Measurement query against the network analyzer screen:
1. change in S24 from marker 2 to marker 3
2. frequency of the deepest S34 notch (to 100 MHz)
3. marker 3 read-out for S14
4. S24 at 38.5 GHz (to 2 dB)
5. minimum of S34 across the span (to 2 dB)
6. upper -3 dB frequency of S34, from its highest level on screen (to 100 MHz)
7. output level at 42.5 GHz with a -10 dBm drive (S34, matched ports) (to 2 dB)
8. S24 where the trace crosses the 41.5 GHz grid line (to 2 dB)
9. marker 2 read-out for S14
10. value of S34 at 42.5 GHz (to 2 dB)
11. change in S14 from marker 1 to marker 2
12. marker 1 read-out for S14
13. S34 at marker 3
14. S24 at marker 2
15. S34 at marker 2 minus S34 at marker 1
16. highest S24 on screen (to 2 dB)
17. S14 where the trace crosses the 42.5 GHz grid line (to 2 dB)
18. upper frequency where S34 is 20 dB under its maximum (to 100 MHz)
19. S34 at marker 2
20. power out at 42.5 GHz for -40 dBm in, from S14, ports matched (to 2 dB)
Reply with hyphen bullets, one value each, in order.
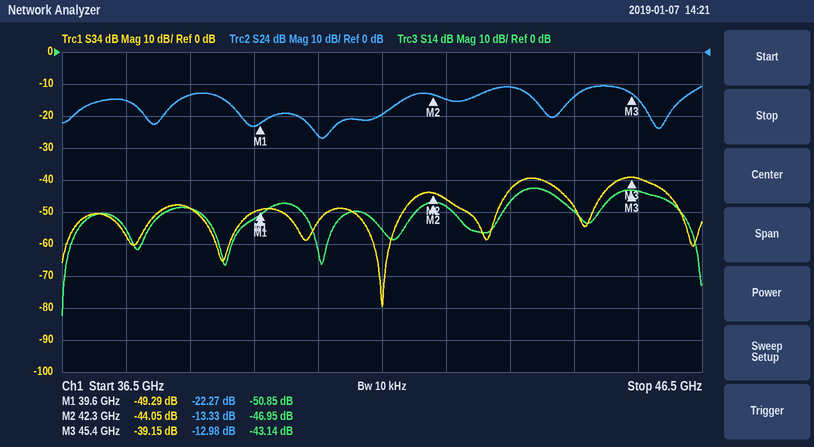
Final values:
- 0.35 dB
- 41.5 GHz
- -43.14 dB
- -14 dB
- -80 dB
- 45.8 GHz
- -56 dBm
- -20 dB
- -46.95 dB
- -46 dB
- 3.90 dB
- -50.85 dB
- -39.15 dB
- -13.33 dB
- 5.24 dB
- -10 dB
- -48 dB
- 46.3 GHz
- -44.05 dB
- -88 dBm
